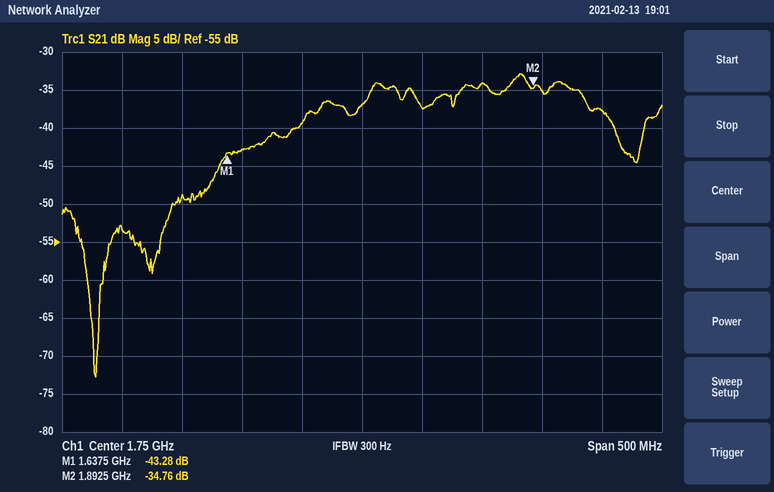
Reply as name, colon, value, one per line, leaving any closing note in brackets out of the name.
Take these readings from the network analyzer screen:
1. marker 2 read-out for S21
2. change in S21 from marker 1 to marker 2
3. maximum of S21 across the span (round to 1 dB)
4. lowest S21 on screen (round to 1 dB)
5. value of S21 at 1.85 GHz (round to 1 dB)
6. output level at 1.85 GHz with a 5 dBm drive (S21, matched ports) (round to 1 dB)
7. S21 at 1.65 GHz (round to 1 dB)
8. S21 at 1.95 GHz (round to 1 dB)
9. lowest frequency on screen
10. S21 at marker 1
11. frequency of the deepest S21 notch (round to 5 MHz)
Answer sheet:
marker 2 read-out for S21: -34.76 dB
change in S21 from marker 1 to marker 2: 8.52 dB
maximum of S21 across the span: -33 dB
lowest S21 on screen: -73 dB
value of S21 at 1.85 GHz: -34 dB
output level at 1.85 GHz with a 5 dBm drive (S21, matched ports): -29 dBm
S21 at 1.65 GHz: -43 dB
S21 at 1.95 GHz: -38 dB
lowest frequency on screen: 1.5 GHz
S21 at marker 1: -43.28 dB
frequency of the deepest S21 notch: 1.530 GHz
